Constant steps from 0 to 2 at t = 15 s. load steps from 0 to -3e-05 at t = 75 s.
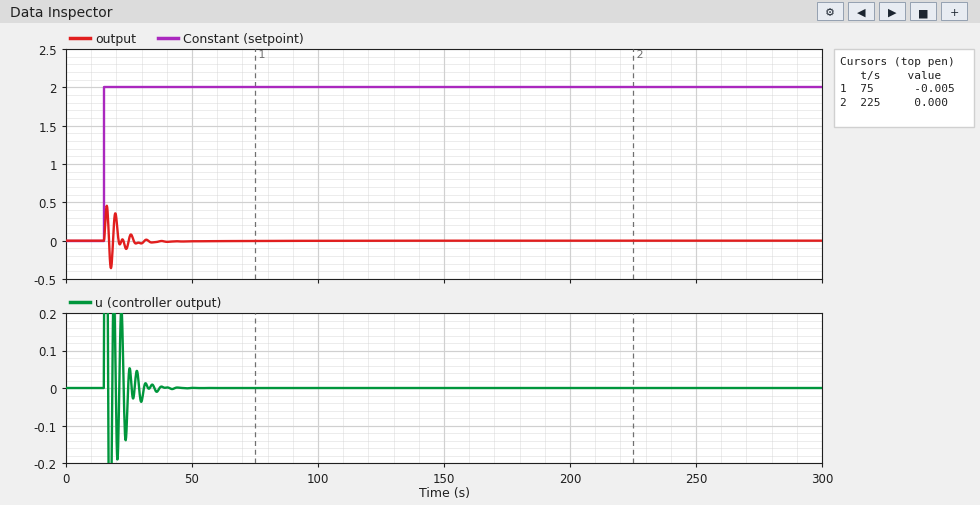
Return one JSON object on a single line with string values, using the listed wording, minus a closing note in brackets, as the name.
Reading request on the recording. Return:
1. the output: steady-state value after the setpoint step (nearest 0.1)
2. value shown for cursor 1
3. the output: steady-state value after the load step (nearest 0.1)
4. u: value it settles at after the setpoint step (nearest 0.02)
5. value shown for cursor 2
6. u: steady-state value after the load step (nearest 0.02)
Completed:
{"the output: steady-state value after the setpoint step": "0.0", "value shown for cursor 1": "-0.005", "the output: steady-state value after the load step": "0.0", "u: value it settles at after the setpoint step": "0.00", "value shown for cursor 2": "0.000", "u: steady-state value after the load step": "0.00"}
